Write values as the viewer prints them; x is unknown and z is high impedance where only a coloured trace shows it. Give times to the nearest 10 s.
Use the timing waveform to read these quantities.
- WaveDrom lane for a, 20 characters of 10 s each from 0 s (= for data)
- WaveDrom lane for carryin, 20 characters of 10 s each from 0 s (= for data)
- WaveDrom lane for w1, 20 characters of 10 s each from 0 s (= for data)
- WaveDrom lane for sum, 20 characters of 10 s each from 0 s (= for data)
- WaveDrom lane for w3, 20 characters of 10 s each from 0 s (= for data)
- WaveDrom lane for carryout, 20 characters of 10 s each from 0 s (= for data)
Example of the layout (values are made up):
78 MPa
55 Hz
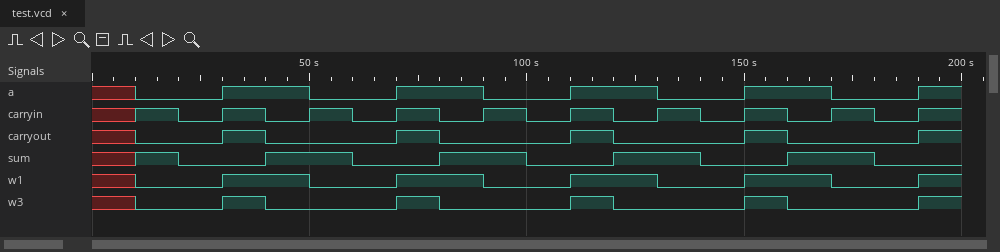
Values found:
{name: 'a', wave: 'x0.1.0.1.0.1.0.1.0.1'}
{name: 'carryin', wave: 'x1010101010101010101'}
{name: 'w1', wave: 'x0.1.0.1.0.1.0.1.0.1'}
{name: 'sum', wave: 'x10.1.0.1.0.1.0.1.0.'}
{name: 'w3', wave: 'x0.10..10..10..10..1'}
{name: 'carryout', wave: 'x0.10..10..10..10..1'}
